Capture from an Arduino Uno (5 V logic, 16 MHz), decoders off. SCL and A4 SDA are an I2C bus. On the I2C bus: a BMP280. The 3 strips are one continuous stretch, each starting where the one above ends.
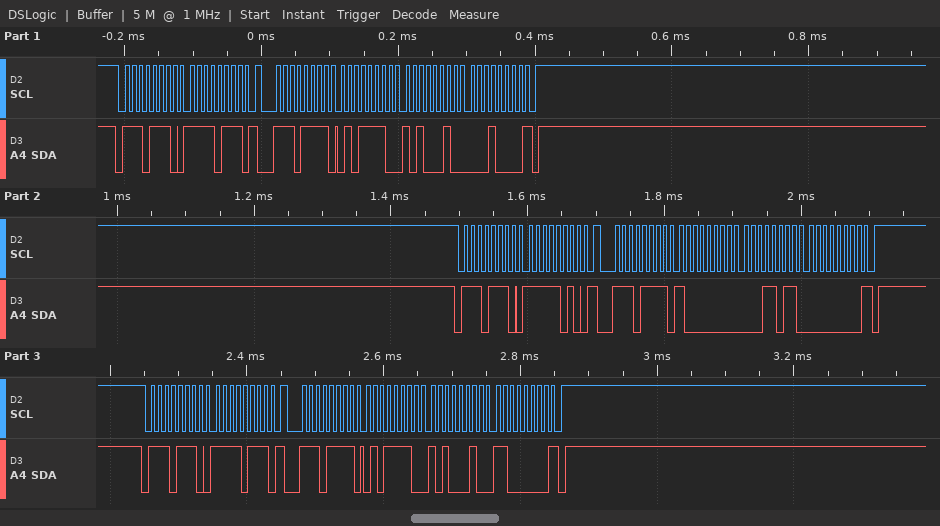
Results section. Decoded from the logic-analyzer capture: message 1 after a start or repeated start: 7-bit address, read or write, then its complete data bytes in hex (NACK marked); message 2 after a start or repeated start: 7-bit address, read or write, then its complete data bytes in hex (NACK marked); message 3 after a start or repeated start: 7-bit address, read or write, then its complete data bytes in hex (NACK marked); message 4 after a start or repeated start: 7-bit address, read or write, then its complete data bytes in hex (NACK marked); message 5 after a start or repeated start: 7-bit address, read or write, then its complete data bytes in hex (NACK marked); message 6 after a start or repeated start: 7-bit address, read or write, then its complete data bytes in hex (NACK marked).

0x77 write: F7
0x77 read: 5E A2 10 NACK
0x77 write: FA
0x77 read: 80 1B 00 NACK
0x77 write: F7
0x77 read: 5E A2 C0 NACK
